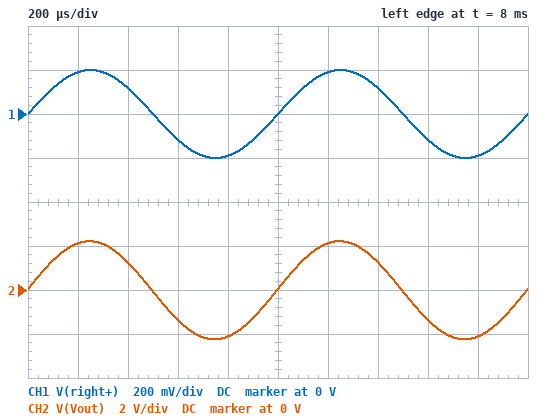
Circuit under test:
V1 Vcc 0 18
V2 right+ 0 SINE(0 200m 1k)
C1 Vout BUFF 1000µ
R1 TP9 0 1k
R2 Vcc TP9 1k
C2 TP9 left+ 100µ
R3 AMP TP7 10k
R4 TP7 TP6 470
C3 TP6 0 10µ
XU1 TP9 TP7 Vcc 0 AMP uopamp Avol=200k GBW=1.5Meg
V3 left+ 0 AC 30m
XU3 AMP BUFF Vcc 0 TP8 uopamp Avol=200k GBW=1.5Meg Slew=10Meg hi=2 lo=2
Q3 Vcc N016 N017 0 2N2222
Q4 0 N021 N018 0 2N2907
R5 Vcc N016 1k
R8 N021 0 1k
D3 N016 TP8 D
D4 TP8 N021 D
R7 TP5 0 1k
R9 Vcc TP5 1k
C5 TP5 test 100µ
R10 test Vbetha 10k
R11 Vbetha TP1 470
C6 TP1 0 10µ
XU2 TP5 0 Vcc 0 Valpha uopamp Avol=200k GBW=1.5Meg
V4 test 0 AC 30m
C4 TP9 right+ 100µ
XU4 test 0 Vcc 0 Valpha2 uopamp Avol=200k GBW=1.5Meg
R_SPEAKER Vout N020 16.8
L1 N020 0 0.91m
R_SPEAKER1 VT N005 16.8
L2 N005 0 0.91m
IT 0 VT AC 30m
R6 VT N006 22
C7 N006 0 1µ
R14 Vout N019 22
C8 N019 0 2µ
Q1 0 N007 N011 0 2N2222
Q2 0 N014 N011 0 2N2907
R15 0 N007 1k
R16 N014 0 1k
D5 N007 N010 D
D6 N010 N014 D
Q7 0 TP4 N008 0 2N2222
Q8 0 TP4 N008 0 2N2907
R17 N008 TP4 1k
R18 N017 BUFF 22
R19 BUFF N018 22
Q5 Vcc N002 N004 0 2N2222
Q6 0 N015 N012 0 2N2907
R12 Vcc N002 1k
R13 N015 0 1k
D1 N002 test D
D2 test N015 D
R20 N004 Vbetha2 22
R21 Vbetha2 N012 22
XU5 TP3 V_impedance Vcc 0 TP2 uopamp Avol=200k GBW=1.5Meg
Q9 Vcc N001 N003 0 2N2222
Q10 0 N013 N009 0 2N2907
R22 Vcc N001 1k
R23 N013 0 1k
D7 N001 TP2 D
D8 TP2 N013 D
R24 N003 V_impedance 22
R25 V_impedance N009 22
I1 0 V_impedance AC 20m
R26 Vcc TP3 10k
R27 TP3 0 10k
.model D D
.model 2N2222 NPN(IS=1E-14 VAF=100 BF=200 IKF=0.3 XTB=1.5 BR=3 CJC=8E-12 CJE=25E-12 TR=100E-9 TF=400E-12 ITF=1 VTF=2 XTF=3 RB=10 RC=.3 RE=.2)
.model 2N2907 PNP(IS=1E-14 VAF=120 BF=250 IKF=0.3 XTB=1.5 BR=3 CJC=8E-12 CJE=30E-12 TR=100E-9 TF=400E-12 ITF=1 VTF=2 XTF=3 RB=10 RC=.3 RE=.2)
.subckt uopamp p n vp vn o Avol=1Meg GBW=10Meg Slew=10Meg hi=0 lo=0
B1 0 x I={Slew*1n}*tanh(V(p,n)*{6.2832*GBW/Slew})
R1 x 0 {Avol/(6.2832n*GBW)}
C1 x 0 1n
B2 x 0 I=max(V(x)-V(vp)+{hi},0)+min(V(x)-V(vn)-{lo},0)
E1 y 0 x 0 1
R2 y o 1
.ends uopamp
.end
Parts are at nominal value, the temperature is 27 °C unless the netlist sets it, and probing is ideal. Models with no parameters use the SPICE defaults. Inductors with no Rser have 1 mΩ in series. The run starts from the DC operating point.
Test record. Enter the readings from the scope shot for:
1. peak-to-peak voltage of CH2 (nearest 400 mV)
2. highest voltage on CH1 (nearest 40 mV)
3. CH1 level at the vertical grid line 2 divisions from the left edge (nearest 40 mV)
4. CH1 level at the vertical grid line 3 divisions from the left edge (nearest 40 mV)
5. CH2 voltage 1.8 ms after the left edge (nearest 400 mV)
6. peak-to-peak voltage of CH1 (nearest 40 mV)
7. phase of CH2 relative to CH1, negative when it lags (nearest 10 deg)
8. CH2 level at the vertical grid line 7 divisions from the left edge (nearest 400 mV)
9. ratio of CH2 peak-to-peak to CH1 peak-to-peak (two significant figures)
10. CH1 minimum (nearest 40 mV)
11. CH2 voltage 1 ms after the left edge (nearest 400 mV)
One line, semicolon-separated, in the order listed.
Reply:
4.4 V; 200 mV; 120 mV; -120 mV; -2.0 V; 400 mV; 0 deg; 1.2 V; 11; -200 mV; 0 V
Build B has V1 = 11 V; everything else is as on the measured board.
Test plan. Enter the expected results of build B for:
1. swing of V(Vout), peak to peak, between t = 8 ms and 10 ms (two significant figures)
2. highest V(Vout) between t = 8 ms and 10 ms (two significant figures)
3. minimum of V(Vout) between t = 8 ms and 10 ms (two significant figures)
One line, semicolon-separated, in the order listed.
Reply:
3.2 V; 1.6 V; -1.6 V
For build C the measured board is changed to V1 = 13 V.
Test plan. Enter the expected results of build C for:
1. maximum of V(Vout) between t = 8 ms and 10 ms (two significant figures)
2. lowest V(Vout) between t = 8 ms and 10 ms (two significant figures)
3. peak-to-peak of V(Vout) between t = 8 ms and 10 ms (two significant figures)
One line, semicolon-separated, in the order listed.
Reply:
2.0 V; -2.0 V; 4.0 V
